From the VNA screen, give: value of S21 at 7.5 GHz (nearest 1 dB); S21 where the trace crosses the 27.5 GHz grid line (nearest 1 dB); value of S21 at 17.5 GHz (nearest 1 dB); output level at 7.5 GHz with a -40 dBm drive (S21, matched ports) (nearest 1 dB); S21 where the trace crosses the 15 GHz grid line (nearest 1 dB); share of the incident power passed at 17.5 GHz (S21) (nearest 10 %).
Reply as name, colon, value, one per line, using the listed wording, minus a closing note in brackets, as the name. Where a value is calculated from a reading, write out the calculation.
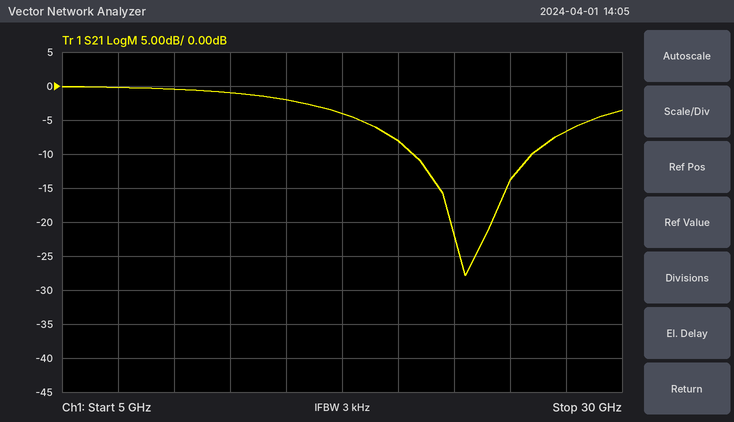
value of S21 at 7.5 GHz: 0 dB
S21 where the trace crosses the 27.5 GHz grid line: -7 dB
value of S21 at 17.5 GHz: -4 dB
output level at 7.5 GHz with a -40 dBm drive (S21, matched ports): -40 dBm + (0 dB) = -40 dBm
S21 where the trace crosses the 15 GHz grid line: -2 dB
share of the incident power passed at 17.5 GHz (S21): 10^(-4/10) ≈ 40 %
